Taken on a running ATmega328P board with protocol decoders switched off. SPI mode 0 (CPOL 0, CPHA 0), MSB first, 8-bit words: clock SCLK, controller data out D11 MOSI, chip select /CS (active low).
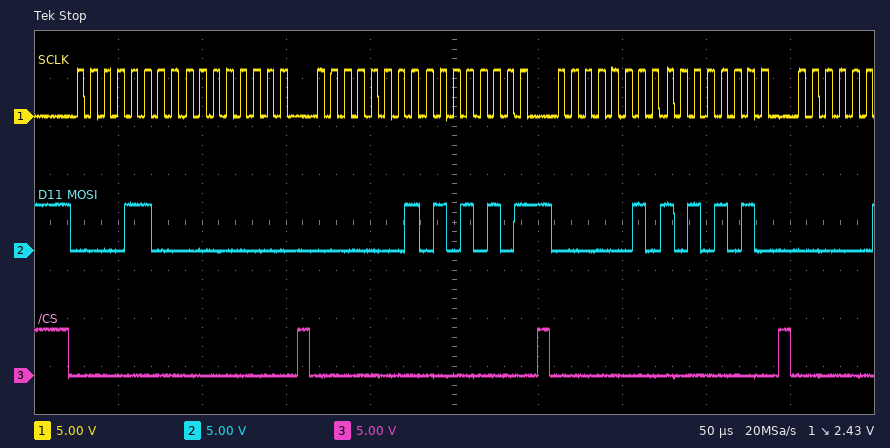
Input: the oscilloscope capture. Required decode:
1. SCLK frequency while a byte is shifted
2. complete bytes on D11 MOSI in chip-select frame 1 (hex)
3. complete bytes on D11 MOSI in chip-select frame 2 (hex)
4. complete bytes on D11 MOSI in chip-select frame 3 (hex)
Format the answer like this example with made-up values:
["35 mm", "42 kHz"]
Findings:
["125 kHz", "0x0C 0x00", "0x01 0x55", "0x02 0xAA"]
